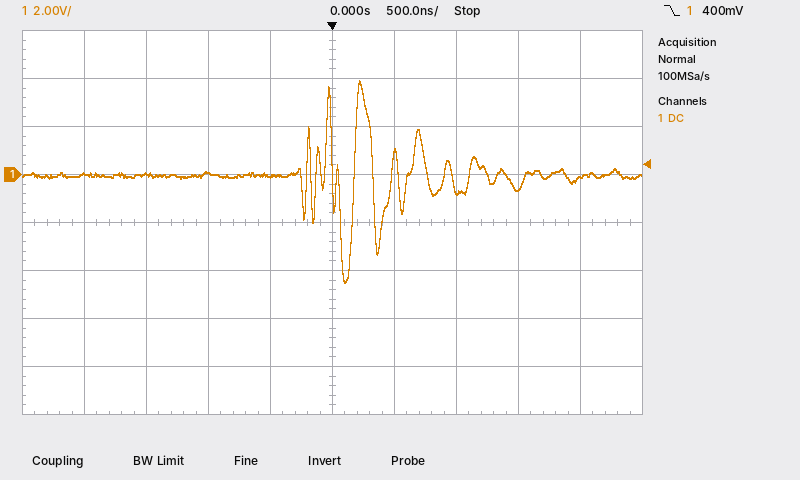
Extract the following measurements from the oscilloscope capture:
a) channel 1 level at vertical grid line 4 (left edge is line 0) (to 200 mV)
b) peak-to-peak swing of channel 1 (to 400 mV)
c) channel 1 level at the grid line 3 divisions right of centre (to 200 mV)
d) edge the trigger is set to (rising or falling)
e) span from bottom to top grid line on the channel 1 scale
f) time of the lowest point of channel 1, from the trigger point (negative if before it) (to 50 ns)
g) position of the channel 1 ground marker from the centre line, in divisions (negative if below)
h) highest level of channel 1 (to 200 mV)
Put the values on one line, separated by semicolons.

0.0 V; 8.4 V; -600 mV; falling; 16 V; +100 ns; +1.0 div; 4.0 V
